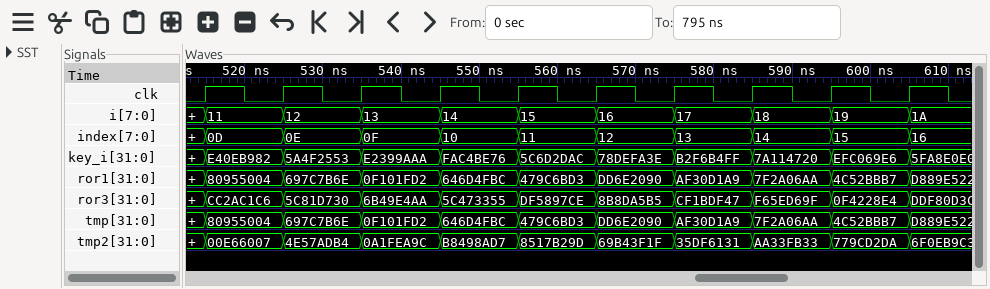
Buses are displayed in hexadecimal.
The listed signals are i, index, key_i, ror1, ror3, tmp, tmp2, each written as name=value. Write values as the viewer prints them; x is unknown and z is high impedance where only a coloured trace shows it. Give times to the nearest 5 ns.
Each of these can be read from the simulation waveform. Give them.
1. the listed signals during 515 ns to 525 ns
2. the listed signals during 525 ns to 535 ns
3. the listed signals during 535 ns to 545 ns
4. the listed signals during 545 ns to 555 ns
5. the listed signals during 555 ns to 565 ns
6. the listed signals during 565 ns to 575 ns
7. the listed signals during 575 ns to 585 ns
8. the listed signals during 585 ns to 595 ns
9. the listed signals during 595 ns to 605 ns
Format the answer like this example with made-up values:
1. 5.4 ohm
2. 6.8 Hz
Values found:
1. i=11, index=0D, key_i=E40EB982, ror1=80955004, ror3=CC2AC1C6, tmp=80955004, tmp2=00E66007
2. i=12, index=0E, key_i=5A4F2553, ror1=697C7B6E, ror3=5C81D730, tmp=697C7B6E, tmp2=4E57ADB4
3. i=13, index=0F, key_i=E2399AAA, ror1=0F101FD2, ror3=6B49E4AA, tmp=0F101FD2, tmp2=0A1FEA9C
4. i=14, index=10, key_i=FAC4BE76, ror1=646D4FBC, ror3=5C473355, tmp=646D4FBC, tmp2=B8498AD7
5. i=15, index=11, key_i=5C6D2DAC, ror1=479C6BD3, ror3=DF5897CE, tmp=479C6BD3, tmp2=8517B29D
6. i=16, index=12, key_i=78DEFA3E, ror1=DD6E2090, ror3=8B8DA5B5, tmp=DD6E2090, tmp2=69B43F1F
7. i=17, index=13, key_i=B2F6B4FF, ror1=AF30D1A9, ror3=CF1BDF47, tmp=AF30D1A9, tmp2=35DF6131
8. i=18, index=14, key_i=7A114720, ror1=7F2A06AA, ror3=F65ED69F, tmp=7F2A06AA, tmp2=AA33FB33
9. i=19, index=15, key_i=EFC069E6, ror1=4C52BBB7, ror3=0F4228E4, tmp=4C52BBB7, tmp2=779CD2DA
